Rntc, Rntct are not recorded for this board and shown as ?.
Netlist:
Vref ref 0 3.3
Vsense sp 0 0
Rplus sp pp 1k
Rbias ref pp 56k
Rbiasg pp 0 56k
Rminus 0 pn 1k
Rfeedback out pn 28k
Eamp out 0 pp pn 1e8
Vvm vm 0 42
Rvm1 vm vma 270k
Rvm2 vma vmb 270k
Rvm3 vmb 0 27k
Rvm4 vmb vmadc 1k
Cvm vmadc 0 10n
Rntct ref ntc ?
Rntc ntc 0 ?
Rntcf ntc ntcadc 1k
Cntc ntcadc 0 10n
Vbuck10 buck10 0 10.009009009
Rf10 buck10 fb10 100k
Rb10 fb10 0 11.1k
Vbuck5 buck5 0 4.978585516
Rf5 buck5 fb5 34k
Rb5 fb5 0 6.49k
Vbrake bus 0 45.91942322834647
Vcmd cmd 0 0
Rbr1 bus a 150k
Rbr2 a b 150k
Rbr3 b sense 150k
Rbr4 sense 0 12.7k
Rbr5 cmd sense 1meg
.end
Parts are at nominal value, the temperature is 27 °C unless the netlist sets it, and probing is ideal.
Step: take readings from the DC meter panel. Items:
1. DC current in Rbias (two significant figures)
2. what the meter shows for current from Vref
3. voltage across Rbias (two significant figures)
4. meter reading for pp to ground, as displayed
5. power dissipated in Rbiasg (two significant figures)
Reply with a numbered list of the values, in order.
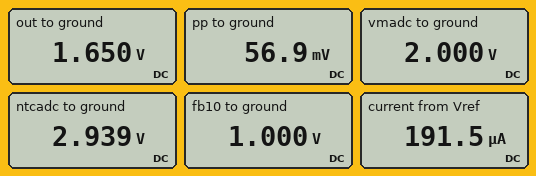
1. 58 µA
2. 191.5 µA
3. 3.2 V
4. 56.9 mV
5. 58 nW
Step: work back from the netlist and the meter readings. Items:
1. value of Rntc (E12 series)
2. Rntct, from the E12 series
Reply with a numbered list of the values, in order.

1. 22 kΩ
2. 2.7 kΩ
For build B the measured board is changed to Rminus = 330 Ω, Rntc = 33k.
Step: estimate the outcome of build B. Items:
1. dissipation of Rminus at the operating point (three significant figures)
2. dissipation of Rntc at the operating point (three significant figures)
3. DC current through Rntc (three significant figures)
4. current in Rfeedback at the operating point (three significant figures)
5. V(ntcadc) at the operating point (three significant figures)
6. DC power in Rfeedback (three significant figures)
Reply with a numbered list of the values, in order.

1. 9.81 µW
2. 282 µW
3. 92.4 µA
4. 172 µA
5. 3.05 V
6. 832 µW
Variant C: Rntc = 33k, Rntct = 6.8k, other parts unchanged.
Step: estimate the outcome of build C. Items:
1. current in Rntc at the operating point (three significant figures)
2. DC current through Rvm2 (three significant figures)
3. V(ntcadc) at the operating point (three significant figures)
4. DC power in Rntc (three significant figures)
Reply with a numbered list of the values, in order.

1. 82.9 µA
2. 74.1 µA
3. 2.74 V
4. 227 µW
